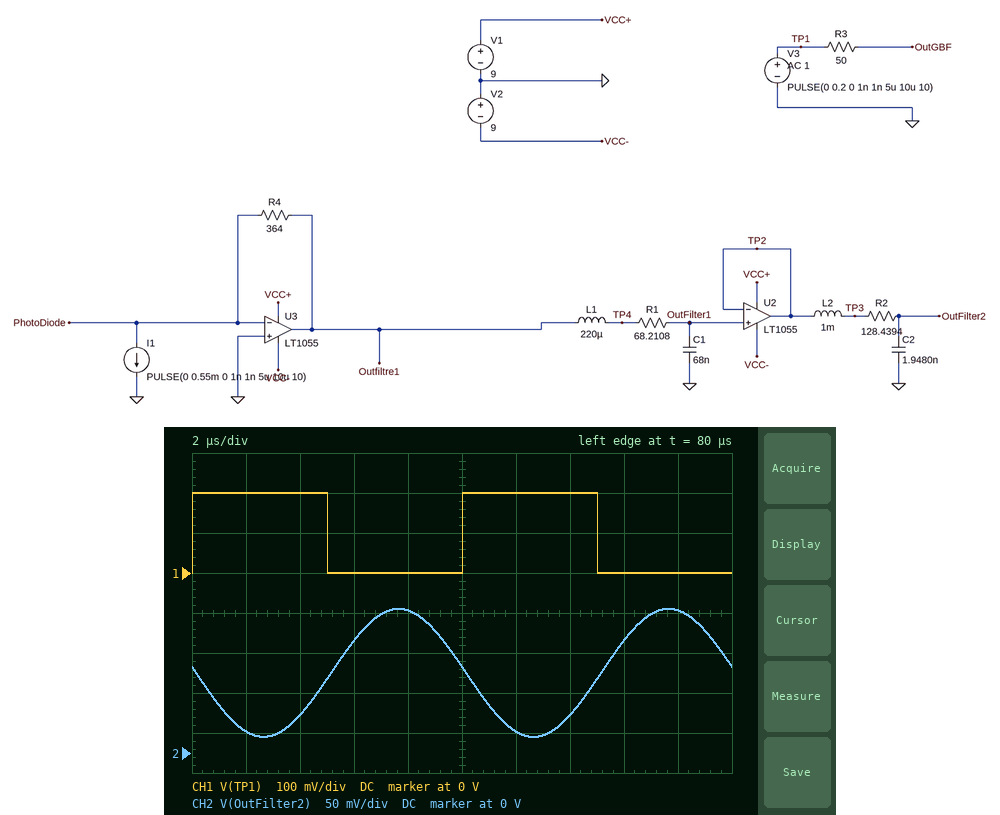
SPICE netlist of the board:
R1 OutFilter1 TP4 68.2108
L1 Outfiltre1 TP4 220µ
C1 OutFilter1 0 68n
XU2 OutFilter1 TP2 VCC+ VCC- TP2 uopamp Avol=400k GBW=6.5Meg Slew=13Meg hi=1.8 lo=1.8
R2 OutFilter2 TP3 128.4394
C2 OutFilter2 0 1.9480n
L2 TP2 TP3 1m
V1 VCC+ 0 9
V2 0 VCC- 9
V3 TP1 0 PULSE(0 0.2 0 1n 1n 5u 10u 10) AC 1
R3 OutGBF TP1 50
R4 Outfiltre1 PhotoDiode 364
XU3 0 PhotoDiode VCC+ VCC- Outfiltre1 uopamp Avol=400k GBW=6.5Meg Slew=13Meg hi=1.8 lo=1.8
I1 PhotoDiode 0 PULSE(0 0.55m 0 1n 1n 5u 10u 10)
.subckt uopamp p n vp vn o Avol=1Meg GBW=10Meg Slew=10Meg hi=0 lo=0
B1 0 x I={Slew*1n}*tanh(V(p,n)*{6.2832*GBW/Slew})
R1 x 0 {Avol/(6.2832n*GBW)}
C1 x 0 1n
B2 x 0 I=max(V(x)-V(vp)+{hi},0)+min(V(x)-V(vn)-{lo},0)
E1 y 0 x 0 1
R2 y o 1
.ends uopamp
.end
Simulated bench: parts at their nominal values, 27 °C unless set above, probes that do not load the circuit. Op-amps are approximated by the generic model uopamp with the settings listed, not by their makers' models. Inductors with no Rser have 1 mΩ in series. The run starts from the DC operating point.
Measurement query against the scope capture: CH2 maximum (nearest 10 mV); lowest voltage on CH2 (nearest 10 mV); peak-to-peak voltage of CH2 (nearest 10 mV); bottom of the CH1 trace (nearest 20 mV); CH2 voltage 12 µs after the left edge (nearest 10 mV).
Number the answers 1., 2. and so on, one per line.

1. 180 mV
2. 20 mV
3. 160 mV
4. 0 V
5. 30 mV
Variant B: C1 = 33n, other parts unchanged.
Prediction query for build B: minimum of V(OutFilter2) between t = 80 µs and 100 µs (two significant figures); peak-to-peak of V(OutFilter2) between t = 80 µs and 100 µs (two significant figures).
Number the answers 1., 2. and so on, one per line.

1. -95 mV
2. 390 mV
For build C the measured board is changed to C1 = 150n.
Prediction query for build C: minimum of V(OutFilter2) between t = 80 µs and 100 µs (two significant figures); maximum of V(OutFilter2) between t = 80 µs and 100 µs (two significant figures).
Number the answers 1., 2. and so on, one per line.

1. 67 mV
2. 130 mV
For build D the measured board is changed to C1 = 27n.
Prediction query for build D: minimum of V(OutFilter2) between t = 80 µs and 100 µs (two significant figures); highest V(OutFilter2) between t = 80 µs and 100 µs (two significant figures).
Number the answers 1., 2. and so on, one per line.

1. -160 mV
2. 360 mV
